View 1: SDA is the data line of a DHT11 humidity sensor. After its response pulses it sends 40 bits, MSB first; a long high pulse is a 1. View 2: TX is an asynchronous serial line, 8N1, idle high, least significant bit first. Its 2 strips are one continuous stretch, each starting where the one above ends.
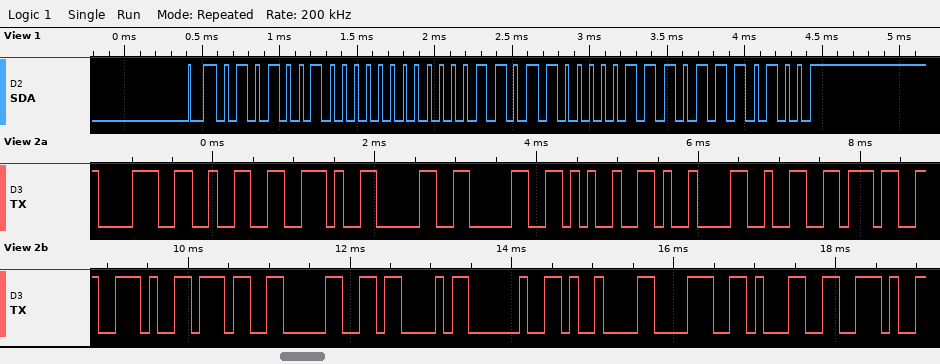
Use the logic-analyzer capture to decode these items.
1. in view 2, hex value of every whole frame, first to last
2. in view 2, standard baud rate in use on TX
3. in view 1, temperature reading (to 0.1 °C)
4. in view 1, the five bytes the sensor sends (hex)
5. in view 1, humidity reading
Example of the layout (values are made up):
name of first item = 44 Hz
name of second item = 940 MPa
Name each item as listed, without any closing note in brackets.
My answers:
in view 2, hex value of every whole frame, first to last = 38 32 2E 30 30 25 09 32 37 2E 37 30 43 20 09 38 31 2E
in view 2, standard baud rate in use on TX = 9600 baud
in view 1, temperature reading = 27.7 °C
in view 1, the five bytes the sensor sends = 52 00 1B 07 74
in view 1, humidity reading = 82 %
